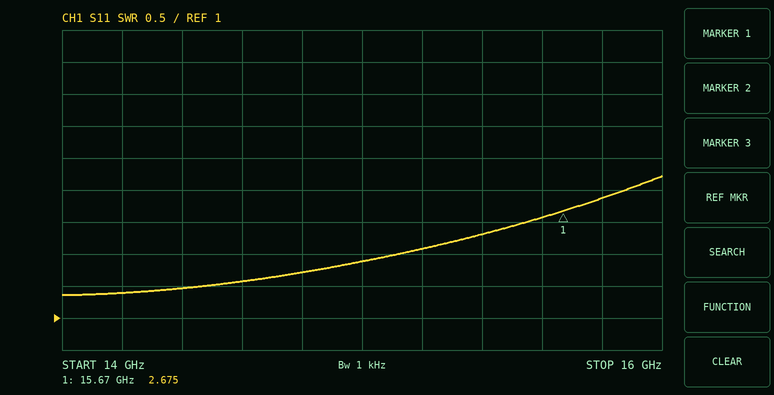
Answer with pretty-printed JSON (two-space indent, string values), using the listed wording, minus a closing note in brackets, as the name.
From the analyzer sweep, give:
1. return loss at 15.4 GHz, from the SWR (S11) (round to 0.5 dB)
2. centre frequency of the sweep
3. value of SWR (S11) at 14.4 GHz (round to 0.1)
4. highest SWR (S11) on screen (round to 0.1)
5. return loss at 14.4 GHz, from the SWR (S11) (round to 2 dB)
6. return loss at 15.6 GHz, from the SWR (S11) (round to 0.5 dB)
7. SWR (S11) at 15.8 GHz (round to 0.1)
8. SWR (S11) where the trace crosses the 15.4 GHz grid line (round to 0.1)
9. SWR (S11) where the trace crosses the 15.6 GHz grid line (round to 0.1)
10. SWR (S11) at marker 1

{
  "return loss at 15.4 GHz, from the SWR (S11)": "8.0 dB",
  "centre frequency of the sweep": "15 GHz",
  "value of SWR (S11) at 14.4 GHz": "1.5",
  "highest SWR (S11) on screen": "3.2",
  "return loss at 14.4 GHz, from the SWR (S11)": "14 dB",
  "return loss at 15.6 GHz, from the SWR (S11)": "7.0 dB",
  "SWR (S11) at 15.8 GHz": "2.9",
  "SWR (S11) where the trace crosses the 15.4 GHz grid line": "2.3",
  "SWR (S11) where the trace crosses the 15.6 GHz grid line": "2.6",
  "SWR (S11) at marker 1": "2.675"
}
